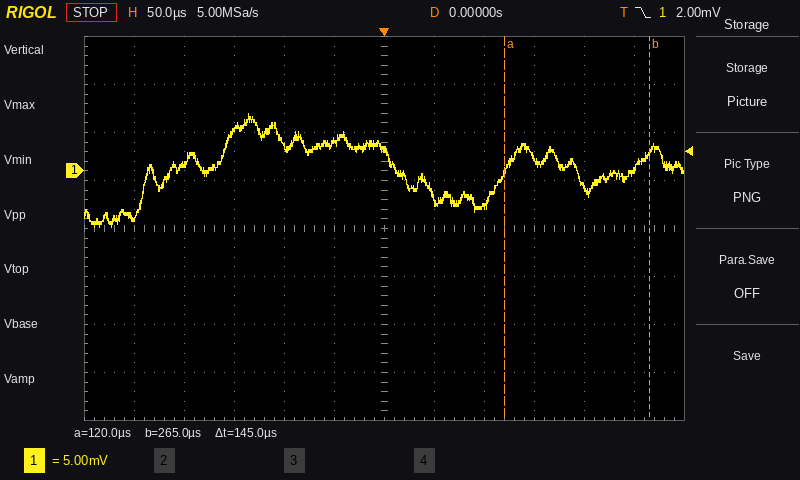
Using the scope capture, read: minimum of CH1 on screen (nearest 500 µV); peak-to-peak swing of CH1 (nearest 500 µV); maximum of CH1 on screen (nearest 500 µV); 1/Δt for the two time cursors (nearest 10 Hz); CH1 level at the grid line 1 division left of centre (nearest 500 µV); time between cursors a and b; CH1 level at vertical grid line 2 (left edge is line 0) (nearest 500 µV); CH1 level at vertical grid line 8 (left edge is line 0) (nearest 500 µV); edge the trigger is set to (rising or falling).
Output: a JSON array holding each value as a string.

["-6.0 mV", "12.0 mV", "6.0 mV", "6.90 kHz", "3.0 mV", "145 µs", "500 µV", "-3.5 mV", "falling"]
